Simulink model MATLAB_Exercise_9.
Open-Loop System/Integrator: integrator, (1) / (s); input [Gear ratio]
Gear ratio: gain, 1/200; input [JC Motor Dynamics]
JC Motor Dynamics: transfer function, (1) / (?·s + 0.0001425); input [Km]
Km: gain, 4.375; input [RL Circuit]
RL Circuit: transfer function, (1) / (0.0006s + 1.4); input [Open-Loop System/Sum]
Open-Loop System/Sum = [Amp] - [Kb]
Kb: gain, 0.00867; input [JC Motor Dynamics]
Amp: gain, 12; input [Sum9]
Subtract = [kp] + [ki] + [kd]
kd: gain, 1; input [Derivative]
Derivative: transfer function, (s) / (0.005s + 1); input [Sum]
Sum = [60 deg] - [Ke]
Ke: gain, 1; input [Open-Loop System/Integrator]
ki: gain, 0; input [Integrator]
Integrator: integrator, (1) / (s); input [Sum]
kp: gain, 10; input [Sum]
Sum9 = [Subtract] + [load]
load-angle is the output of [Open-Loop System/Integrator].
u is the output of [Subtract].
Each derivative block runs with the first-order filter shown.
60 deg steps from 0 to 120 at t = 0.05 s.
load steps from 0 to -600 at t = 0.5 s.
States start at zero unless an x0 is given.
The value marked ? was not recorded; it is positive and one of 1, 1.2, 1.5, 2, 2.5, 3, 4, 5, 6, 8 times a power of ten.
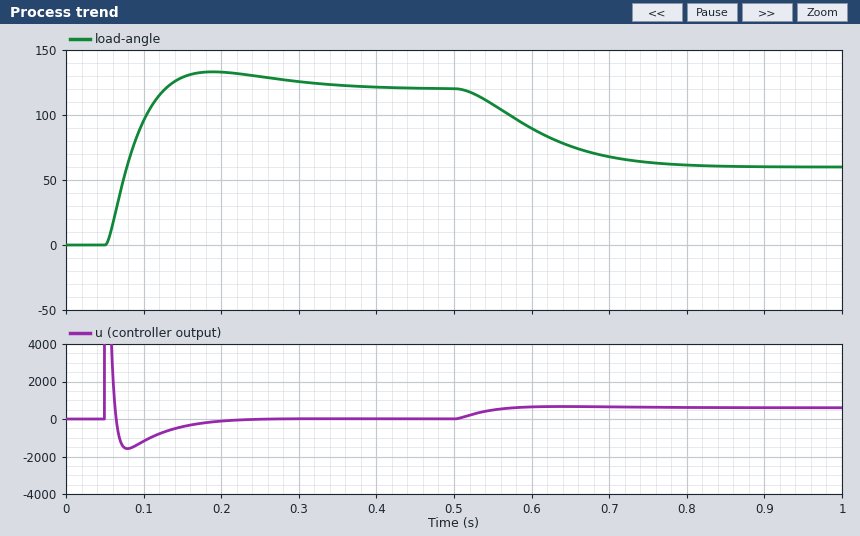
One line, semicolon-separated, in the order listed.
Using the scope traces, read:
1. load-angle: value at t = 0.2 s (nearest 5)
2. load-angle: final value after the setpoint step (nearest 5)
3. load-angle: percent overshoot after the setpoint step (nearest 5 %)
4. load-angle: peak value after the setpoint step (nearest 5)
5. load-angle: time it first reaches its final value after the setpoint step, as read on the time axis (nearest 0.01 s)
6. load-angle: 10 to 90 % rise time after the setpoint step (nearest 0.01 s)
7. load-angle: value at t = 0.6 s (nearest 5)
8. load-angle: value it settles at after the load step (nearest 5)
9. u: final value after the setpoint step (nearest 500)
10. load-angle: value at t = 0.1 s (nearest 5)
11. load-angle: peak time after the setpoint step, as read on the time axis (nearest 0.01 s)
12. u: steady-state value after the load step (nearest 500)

135; 120; 10 %; 135; 0.13 s; 0.05 s; 90; 60; 0; 95; 0.19 s; 500
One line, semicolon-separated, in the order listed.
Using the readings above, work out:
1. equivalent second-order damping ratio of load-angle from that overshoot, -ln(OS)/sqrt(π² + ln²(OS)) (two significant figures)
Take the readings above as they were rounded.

0.59
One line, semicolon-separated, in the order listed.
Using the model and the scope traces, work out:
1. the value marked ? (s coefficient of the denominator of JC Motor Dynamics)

0.008
